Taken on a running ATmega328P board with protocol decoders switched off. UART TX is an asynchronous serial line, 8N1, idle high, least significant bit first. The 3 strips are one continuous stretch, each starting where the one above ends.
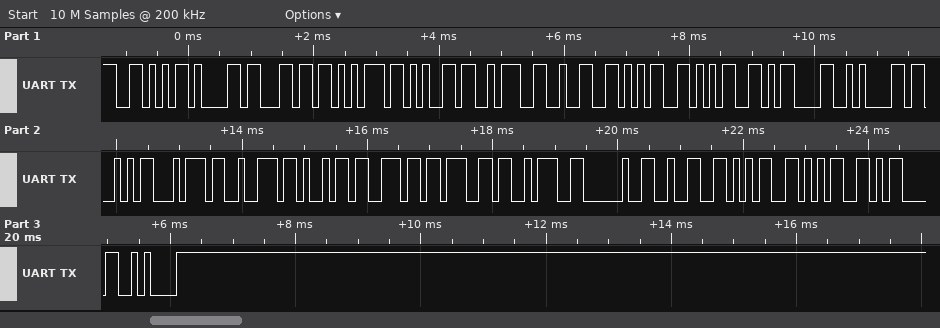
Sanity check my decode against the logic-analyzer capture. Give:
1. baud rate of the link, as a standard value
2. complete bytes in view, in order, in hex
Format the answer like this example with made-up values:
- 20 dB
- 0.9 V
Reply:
- 9600 baud
- 56 61 6C 75 65 3A 32 35 35 0D 0A 53 74 72 69 6E 67 3A 20 32 35 35 0D 0A
